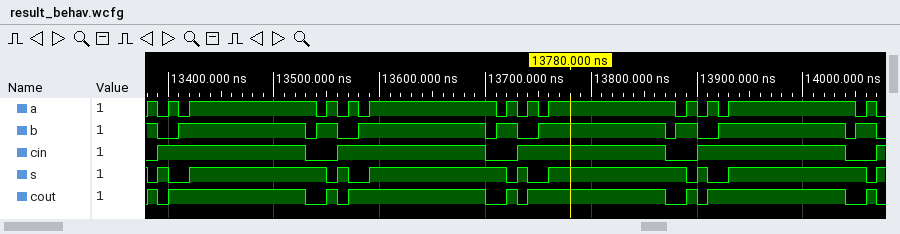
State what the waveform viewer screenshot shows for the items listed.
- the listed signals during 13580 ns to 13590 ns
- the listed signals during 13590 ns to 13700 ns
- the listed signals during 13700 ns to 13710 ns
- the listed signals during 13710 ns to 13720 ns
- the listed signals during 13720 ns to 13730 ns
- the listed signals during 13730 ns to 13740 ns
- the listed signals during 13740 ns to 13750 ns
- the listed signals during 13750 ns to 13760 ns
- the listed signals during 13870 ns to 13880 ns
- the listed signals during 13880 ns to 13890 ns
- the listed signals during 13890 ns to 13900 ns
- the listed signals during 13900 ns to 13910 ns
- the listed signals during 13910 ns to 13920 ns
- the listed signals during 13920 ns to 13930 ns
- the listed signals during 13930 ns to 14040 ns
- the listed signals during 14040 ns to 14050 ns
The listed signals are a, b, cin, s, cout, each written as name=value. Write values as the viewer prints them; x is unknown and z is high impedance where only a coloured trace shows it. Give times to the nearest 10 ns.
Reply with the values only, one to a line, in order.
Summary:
a=0, b=1, cin=1, s=0, cout=1
a=1, b=1, cin=1, s=1, cout=1
a=1, b=0, cin=0, s=1, cout=0
a=0, b=1, cin=0, s=1, cout=0
a=1, b=1, cin=0, s=0, cout=1
a=0, b=0, cin=1, s=1, cout=0
a=1, b=0, cin=1, s=0, cout=1
a=0, b=1, cin=1, s=0, cout=1
a=1, b=0, cin=0, s=1, cout=0
a=0, b=1, cin=0, s=1, cout=0
a=1, b=1, cin=0, s=0, cout=1
a=0, b=0, cin=1, s=1, cout=0
a=1, b=0, cin=1, s=0, cout=1
a=0, b=1, cin=1, s=0, cout=1
a=1, b=1, cin=1, s=1, cout=1
a=1, b=0, cin=0, s=1, cout=0
